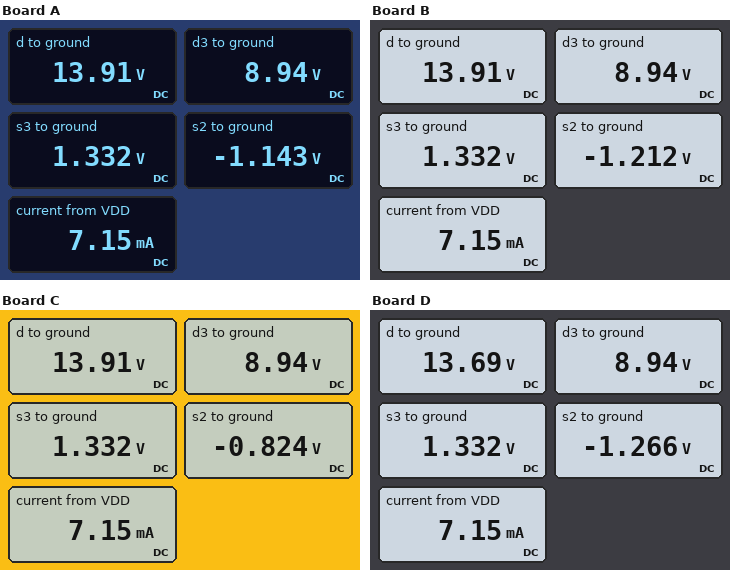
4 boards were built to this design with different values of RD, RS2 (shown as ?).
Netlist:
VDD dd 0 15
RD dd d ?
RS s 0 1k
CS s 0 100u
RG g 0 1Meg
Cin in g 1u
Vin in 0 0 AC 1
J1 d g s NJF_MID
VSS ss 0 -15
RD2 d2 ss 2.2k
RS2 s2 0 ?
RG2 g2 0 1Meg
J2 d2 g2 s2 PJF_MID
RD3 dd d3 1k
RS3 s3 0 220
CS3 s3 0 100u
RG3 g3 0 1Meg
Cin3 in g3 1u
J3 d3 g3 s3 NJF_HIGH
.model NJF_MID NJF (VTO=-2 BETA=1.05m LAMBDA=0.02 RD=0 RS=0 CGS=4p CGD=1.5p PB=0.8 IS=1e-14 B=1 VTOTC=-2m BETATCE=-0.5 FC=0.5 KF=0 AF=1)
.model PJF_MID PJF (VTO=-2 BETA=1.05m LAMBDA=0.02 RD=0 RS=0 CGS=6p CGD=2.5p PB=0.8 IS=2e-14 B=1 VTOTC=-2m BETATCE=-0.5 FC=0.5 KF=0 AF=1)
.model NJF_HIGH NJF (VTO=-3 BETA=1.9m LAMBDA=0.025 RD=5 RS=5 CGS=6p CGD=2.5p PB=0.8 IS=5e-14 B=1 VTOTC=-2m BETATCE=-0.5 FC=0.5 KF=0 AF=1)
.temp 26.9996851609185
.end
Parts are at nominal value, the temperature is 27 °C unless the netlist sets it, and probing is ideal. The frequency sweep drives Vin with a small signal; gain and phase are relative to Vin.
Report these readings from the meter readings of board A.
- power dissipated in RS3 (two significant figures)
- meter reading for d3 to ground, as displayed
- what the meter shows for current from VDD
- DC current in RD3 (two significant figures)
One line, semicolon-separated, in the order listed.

8.1 mW; 8.94 V; 7.15 mA; 6.1 mA
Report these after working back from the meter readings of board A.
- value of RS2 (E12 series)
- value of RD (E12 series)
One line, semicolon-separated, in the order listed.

1.2 kΩ; 1 kΩ
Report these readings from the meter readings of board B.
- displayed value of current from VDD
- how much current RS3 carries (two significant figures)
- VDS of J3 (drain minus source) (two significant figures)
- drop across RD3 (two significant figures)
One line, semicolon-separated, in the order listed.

7.15 mA; 6.1 mA; 7.6 V; 6.1 V
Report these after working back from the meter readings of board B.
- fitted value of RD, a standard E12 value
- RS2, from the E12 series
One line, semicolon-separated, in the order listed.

1 kΩ; 1.5 kΩ
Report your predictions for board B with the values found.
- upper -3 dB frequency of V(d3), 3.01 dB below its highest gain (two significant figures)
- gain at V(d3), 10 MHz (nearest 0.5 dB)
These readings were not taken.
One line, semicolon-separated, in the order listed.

260 MHz; 16.0 dB
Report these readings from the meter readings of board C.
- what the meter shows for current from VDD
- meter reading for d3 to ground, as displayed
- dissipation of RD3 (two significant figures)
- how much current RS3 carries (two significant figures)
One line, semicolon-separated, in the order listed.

7.15 mA; 8.94 V; 37 mW; 6.1 mA
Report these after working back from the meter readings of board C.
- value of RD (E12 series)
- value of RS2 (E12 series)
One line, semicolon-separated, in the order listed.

1 kΩ; 470 Ω
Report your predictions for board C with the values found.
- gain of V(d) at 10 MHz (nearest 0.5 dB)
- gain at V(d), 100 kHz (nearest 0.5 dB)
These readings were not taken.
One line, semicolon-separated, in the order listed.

7.5 dB; 7.5 dB
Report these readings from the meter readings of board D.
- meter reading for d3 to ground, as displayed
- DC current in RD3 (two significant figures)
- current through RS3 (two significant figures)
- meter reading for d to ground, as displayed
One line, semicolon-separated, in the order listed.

8.94 V; 6.1 mA; 6.1 mA; 13.69 V
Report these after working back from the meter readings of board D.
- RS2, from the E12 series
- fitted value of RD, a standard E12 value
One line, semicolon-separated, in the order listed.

1.8 kΩ; 1.2 kΩ
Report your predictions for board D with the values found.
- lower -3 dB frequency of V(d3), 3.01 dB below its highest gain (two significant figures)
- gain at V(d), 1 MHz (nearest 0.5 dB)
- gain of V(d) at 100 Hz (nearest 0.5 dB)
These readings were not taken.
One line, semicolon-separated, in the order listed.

14 Hz; 9.0 dB; 9.0 dB
